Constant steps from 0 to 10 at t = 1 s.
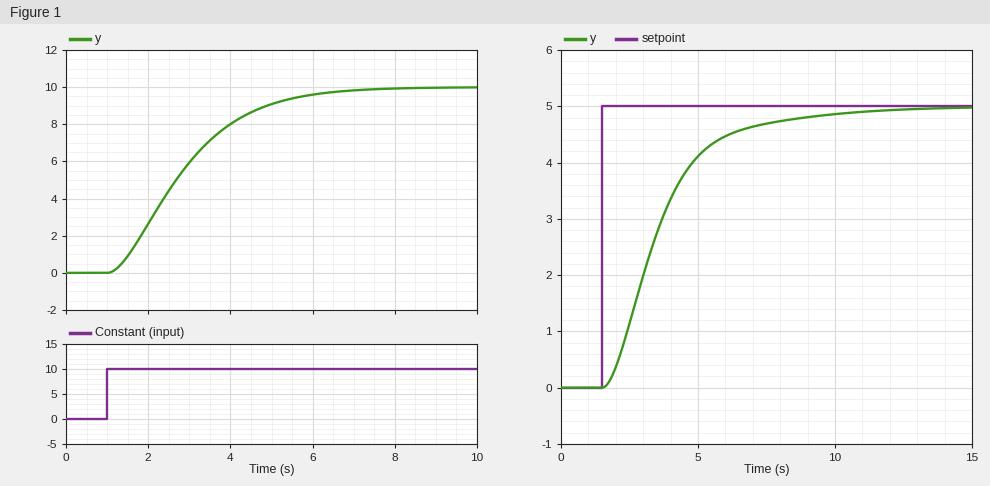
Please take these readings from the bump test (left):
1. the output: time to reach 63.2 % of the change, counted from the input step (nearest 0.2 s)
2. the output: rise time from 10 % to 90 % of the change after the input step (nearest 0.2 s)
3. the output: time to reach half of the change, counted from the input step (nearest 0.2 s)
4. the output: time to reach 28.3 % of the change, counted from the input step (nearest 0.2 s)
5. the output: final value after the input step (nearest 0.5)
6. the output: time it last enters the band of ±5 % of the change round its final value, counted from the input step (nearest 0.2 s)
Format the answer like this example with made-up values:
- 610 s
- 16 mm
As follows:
- 2.2 s
- 3.4 s
- 1.6 s
- 1.0 s
- 10.0
- 4.8 s
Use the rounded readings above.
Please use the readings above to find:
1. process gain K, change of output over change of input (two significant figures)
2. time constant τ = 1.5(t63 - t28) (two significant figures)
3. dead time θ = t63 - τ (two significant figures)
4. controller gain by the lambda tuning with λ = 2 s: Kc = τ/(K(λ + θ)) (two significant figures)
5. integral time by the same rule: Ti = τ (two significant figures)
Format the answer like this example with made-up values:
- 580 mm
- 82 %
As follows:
- 1.0
- 1.8 s
- 0.40 s
- 0.75
- 1.8 s
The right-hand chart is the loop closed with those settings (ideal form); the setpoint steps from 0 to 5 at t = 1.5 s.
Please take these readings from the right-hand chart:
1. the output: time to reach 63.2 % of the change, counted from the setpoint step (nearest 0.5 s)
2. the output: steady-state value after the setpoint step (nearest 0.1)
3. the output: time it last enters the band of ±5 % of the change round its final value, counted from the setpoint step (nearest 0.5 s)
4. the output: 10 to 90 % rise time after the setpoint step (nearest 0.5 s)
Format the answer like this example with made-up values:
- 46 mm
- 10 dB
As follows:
- 2.5 s
- 5.0
- 6.5 s
- 4.0 s
